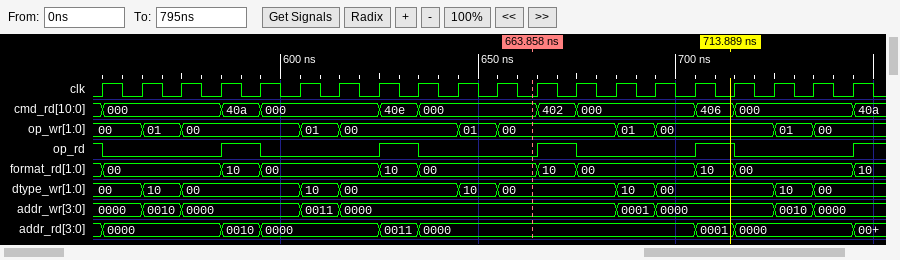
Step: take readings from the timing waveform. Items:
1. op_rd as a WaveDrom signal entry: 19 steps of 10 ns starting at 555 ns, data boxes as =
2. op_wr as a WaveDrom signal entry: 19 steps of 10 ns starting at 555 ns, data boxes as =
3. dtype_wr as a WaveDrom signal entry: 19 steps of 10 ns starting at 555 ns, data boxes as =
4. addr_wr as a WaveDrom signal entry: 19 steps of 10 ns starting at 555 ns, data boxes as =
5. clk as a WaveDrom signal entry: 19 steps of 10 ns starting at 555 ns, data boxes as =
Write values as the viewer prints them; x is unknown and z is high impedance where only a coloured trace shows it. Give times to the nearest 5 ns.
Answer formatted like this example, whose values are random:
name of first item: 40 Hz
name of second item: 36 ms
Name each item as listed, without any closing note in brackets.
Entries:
op_rd as a WaveDrom signal entry: 19 steps of 10 ns starting at 555 ns, data boxes as =: {name: 'op_rd', wave: '0..10..10..10..10..'}
op_wr as a WaveDrom signal entry: 19 steps of 10 ns starting at 555 ns, data boxes as =: {name: 'op_wr', wave: '===..==..==..==..==', data: '00 01 00 01 00 01 00 01 00 01 00'}
dtype_wr as a WaveDrom signal entry: 19 steps of 10 ns starting at 555 ns, data boxes as =: {name: 'dtype_wr', wave: '===..==..==..==..==', data: '00 10 00 10 00 10 00 10 00 10 00'}
addr_wr as a WaveDrom signal entry: 19 steps of 10 ns starting at 555 ns, data boxes as =: {name: 'addr_wr', wave: '===..==......==..==', data: '0000 0010 0000 0011 0000 0001 0000 0010 0000'}
clk as a WaveDrom signal entry: 19 steps of 10 ns starting at 555 ns, data boxes as =: {name: 'clk', wave: 'p..................'}
